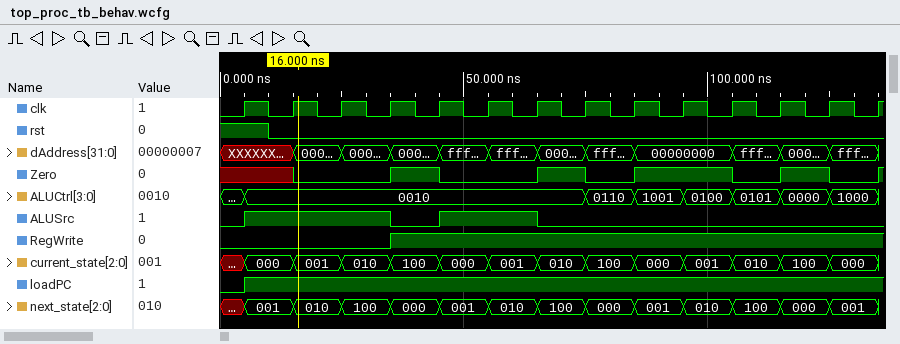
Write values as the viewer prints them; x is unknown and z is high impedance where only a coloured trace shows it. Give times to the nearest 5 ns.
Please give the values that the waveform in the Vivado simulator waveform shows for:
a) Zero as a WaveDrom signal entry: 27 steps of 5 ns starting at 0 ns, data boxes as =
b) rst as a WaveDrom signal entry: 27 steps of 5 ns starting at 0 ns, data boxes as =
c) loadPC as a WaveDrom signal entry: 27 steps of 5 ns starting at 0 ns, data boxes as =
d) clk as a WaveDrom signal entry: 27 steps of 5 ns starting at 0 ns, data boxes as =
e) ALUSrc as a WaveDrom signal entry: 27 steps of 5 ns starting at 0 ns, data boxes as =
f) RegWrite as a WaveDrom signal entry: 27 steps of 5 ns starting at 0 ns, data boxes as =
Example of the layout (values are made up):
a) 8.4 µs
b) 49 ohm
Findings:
a) {name: 'Zero', wave: 'x..0...1.0...1.0.1...0.1.0.'}
b) {name: 'rst', wave: '1.0........................'}
c) {name: 'loadPC', wave: '01.........................'}
d) {name: 'clk', wave: '010101010101010101010101010'}
e) {name: 'ALUSrc', wave: '01.....0.1...0.............'}
f) {name: 'RegWrite', wave: '0......1...................'}
